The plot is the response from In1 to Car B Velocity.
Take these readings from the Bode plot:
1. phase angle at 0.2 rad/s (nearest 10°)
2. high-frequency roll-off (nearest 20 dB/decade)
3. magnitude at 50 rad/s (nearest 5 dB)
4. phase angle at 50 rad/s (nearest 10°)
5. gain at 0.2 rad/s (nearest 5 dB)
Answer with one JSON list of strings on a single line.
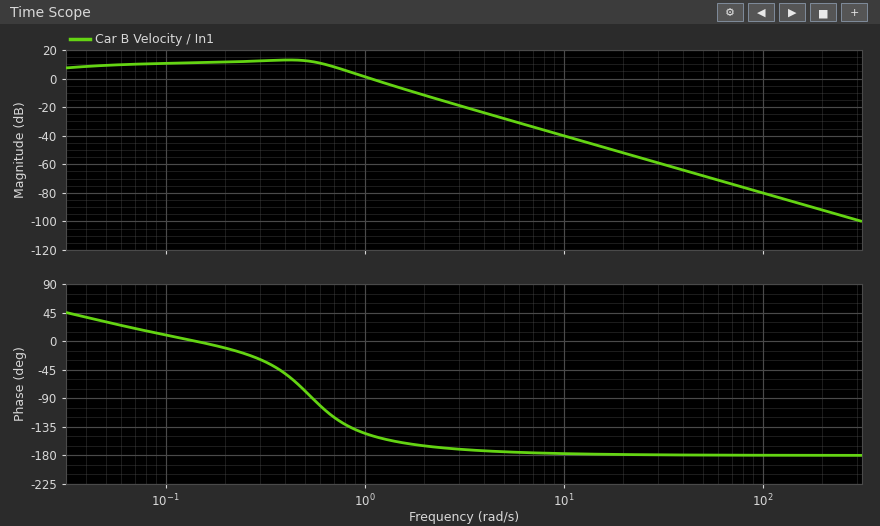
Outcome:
["-10°", "-40 dB/decade", "-70 dB", "-180°", "10 dB"]
